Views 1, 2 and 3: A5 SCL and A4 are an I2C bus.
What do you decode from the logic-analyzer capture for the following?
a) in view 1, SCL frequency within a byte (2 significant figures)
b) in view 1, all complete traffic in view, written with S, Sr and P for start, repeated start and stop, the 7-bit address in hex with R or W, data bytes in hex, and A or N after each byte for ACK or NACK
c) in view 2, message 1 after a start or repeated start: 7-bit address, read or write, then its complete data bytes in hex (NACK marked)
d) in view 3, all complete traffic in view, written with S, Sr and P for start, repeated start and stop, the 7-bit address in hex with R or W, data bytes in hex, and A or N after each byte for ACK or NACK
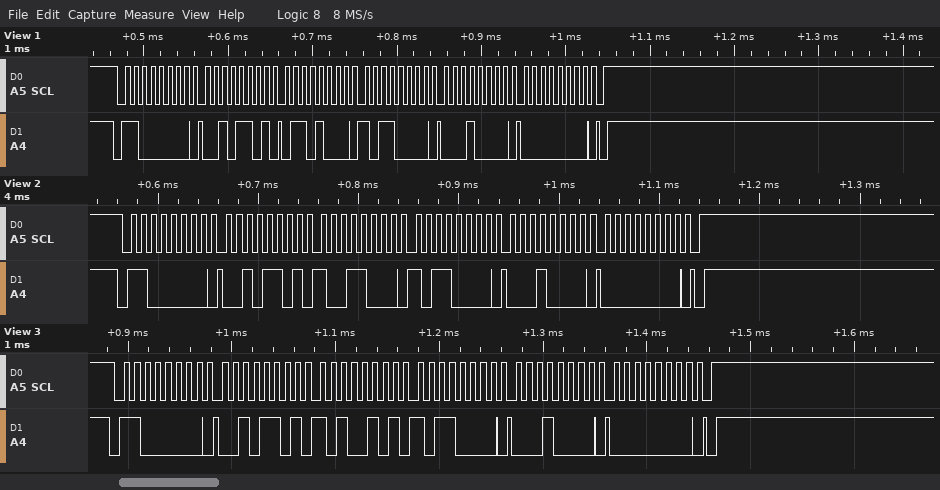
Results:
100 kHz
S 60W A 2D A 68 A B0 A 10 A 00 A P
0x60 write: 2D 98 B0 10 00
S 60W A 2D A A5 A B0 A 10 A 00 A P
